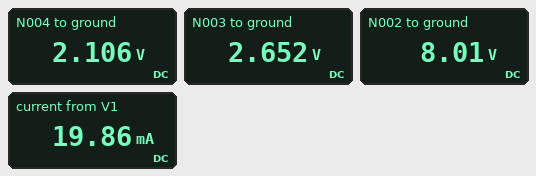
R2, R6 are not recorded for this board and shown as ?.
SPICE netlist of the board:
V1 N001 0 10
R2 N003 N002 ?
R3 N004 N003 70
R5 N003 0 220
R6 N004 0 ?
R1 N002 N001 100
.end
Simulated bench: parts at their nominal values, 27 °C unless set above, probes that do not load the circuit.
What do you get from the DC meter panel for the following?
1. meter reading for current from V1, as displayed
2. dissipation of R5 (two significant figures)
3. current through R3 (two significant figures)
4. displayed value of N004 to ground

19.86 mA
32 mW
7.8 mA
2.106 V
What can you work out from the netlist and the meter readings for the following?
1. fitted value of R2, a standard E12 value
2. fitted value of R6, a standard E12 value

270 Ω
270 Ω
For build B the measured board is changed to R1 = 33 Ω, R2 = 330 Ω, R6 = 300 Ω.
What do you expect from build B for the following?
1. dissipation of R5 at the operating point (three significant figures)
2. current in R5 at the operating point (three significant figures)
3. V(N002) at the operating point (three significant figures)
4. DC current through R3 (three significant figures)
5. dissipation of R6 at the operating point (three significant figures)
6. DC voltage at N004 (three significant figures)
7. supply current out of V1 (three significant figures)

34.5 mW
12.5 mA
9.34 V
7.44 mA
16.6 mW
2.23 V
20.0 mA
